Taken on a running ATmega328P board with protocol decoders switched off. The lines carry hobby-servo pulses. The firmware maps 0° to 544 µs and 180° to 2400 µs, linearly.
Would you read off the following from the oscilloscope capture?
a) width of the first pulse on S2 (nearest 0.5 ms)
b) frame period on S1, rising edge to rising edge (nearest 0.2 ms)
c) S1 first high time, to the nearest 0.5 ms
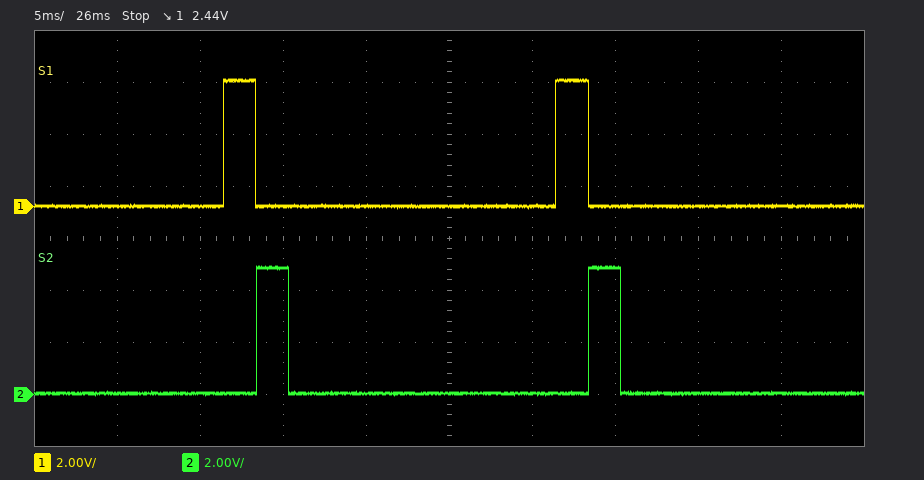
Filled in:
2.0 ms
20.0 ms
2.0 ms
